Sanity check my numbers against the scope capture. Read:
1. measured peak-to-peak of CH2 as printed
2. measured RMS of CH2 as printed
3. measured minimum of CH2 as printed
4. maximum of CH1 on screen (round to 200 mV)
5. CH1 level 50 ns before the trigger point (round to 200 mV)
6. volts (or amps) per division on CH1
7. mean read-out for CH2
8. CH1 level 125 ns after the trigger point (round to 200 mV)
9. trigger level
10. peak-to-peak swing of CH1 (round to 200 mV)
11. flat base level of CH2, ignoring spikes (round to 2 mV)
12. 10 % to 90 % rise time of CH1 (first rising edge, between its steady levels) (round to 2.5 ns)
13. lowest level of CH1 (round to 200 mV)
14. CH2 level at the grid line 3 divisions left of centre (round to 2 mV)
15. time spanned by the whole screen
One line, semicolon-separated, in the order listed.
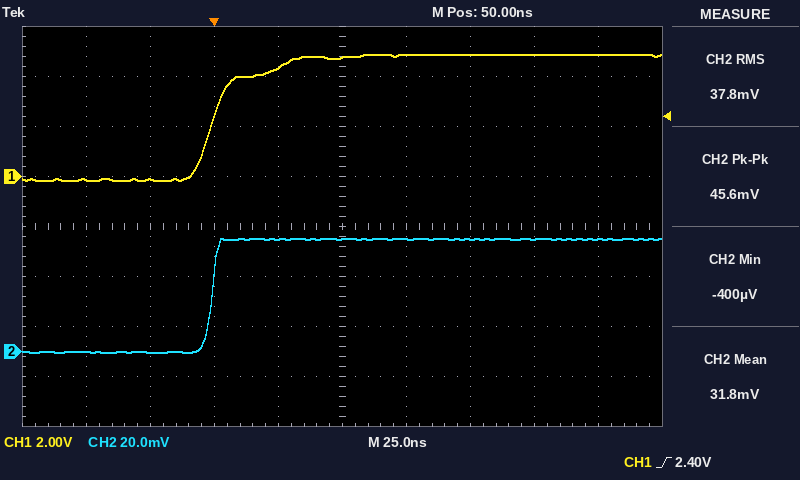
45.6 mV; 37.8 mV; -400 µV; 4.8 V; -200 mV; 2 V; 31.8 mV; 4.8 V; 2.40 V; 5.0 V; 0 mV; 32.5 ns; -200 mV; 0 mV; 250 ns
